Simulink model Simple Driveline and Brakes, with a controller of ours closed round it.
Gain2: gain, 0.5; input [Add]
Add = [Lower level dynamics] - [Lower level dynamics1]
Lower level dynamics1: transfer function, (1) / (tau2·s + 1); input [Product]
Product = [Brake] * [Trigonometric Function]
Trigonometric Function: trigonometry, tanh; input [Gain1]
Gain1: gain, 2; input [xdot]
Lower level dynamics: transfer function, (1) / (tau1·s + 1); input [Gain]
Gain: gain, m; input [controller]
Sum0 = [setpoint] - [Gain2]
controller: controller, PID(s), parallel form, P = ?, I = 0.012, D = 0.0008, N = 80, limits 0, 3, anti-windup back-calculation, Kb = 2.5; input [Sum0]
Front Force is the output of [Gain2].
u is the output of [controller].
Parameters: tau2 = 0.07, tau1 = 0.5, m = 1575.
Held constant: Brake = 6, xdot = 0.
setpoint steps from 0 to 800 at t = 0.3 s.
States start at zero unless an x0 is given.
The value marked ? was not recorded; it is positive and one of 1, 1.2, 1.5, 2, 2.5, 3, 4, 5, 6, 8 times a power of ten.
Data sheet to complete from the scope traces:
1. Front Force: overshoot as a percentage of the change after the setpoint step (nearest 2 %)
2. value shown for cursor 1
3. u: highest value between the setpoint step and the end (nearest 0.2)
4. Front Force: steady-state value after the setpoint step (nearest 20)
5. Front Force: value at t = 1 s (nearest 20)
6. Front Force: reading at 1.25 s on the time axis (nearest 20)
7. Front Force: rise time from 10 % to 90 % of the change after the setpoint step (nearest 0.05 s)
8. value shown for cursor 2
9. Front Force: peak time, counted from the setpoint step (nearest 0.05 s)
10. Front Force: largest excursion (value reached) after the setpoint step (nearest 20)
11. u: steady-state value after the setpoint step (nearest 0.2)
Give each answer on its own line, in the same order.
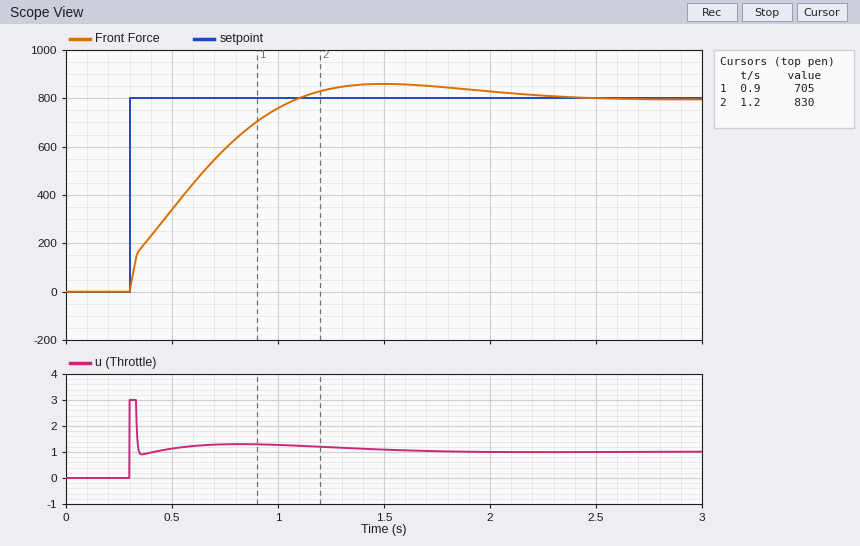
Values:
8 %
705
3.0
800
760
840
0.60 s
830
1.20 s
860
1.0
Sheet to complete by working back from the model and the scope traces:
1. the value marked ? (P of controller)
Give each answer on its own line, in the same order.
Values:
0.004
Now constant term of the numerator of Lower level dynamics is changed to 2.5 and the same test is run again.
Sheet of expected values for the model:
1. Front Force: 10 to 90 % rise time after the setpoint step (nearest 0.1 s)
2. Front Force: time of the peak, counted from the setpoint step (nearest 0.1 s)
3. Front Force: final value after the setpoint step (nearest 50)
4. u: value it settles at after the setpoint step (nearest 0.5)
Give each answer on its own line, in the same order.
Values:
0.5 s
1.0 s
800
0.5
